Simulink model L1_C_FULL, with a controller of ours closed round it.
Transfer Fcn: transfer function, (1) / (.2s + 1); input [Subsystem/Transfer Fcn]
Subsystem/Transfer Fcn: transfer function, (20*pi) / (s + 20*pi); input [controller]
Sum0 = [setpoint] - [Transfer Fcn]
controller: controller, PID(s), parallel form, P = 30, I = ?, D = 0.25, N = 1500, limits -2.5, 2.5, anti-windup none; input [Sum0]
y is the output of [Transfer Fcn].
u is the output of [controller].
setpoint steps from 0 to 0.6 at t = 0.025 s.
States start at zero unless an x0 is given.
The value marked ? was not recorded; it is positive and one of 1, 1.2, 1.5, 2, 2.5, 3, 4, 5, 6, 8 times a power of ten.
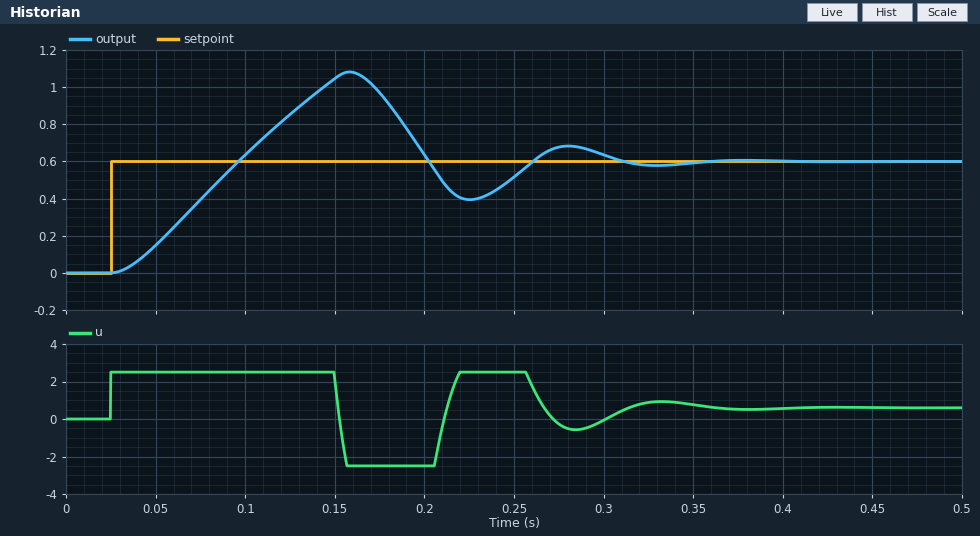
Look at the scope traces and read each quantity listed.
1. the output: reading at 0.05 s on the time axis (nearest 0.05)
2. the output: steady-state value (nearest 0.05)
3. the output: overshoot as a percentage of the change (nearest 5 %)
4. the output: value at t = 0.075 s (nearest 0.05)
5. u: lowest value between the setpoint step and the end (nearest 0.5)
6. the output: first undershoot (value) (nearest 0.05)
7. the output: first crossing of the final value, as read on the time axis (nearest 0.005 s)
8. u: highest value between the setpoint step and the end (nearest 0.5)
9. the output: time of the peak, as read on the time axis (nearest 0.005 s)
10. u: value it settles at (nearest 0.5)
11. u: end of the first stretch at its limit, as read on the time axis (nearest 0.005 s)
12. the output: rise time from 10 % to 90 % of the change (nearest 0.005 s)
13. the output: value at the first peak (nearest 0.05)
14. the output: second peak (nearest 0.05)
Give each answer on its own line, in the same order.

0.15
0.60
80 %
0.40
-2.5
0.40
0.095 s
2.5
0.160 s
0.5
0.150 s
0.050 s
1.10
0.70
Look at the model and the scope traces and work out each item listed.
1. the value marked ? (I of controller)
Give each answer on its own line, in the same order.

1500
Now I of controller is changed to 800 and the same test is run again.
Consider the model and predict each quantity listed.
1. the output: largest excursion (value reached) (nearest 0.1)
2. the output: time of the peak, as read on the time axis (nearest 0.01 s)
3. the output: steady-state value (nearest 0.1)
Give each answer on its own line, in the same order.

1.0
0.15 s
0.6
